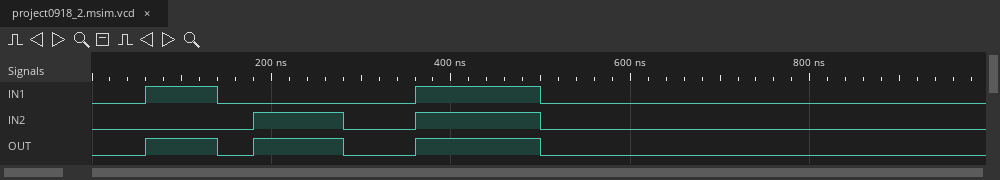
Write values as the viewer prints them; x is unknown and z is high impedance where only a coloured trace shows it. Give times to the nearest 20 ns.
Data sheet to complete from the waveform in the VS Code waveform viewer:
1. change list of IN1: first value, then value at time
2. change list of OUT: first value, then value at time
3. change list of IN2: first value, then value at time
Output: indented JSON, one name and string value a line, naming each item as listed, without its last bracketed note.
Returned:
{
  "change list of IN1: first value, then value at time": "0, 1 at 60 ns, 0 at 140 ns, 1 at 360 ns, 0 at 500 ns",
  "change list of OUT: first value, then value at time": "0, 1 at 60 ns, 0 at 140 ns, 1 at 180 ns, 0 at 280 ns, 1 at 360 ns, 0 at 500 ns",
  "change list of IN2: first value, then value at time": "0, 1 at 180 ns, 0 at 280 ns, 1 at 360 ns, 0 at 500 ns"
}
